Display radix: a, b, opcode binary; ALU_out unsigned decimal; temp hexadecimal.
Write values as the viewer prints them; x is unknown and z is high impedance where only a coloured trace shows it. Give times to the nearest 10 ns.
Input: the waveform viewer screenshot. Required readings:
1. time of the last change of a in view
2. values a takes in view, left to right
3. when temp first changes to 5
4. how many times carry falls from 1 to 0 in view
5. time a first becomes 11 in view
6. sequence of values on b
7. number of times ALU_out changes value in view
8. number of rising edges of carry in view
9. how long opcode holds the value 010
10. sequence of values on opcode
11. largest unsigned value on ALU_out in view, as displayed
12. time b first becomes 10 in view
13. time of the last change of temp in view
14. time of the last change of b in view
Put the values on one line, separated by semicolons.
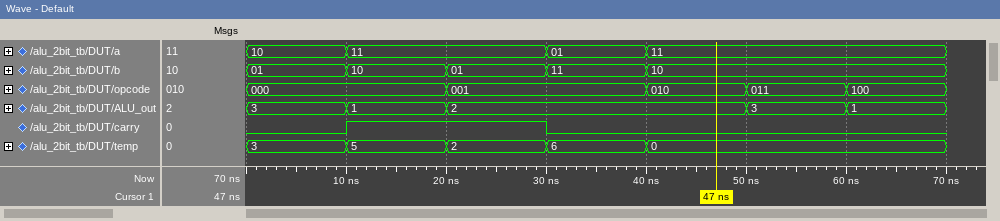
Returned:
40 ns; 10, 11, 01, 11; 10 ns; 1; 10 ns; 01, 10, 01, 11, 10; 4; 1; 10 ns; 000, 001, 010, 011, 100; 3; 10 ns; 40 ns; 40 ns
